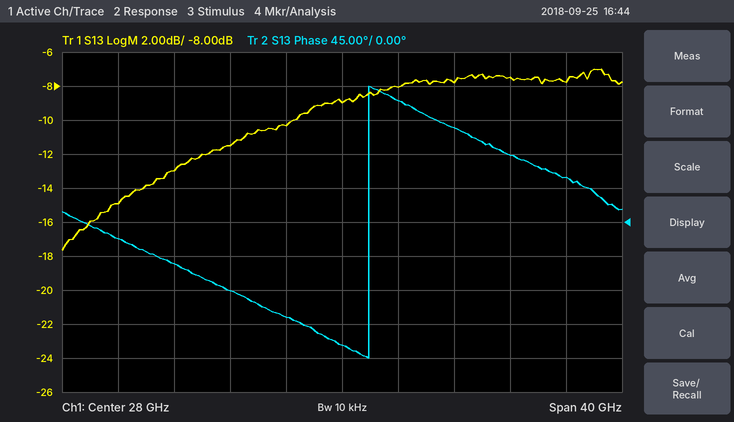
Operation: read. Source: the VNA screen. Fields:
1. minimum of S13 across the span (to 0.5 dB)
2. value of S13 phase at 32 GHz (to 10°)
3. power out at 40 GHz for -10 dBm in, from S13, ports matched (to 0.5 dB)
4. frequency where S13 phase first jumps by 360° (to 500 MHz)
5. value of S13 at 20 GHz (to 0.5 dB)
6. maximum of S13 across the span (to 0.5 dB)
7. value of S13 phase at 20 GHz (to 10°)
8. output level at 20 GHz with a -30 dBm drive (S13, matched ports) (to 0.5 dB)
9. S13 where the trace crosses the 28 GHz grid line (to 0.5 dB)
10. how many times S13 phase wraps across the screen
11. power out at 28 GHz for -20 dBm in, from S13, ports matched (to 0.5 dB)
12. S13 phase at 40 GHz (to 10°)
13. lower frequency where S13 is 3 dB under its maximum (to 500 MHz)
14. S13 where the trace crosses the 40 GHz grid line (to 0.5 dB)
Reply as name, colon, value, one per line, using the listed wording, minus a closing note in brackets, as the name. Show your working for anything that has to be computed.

minimum of S13 across the span: -17.5 dB
value of S13 phase at 32 GHz: 160°
power out at 40 GHz for -10 dBm in, from S13, ports matched: -10 dBm + (-7.5 dB) = -17.5 dBm
frequency where S13 phase first jumps by 360°: 30.0 GHz
value of S13 at 20 GHz: -11.5 dB
maximum of S13 across the span: -7.0 dB
value of S13 phase at 20 GHz: -90°
output level at 20 GHz with a -30 dBm drive (S13, matched ports): -30 dBm + (-11.5 dB) = -41.5 dBm
S13 where the trace crosses the 28 GHz grid line: -9.0 dB
how many times S13 phase wraps across the screen: 1
power out at 28 GHz for -20 dBm in, from S13, ports matched: -20 dBm + (-9.0 dB) = -29.0 dBm
S13 phase at 40 GHz: 90°
lower frequency where S13 is 3 dB under its maximum: 24.5 GHz
S13 where the trace crosses the 40 GHz grid line: -7.5 dB
